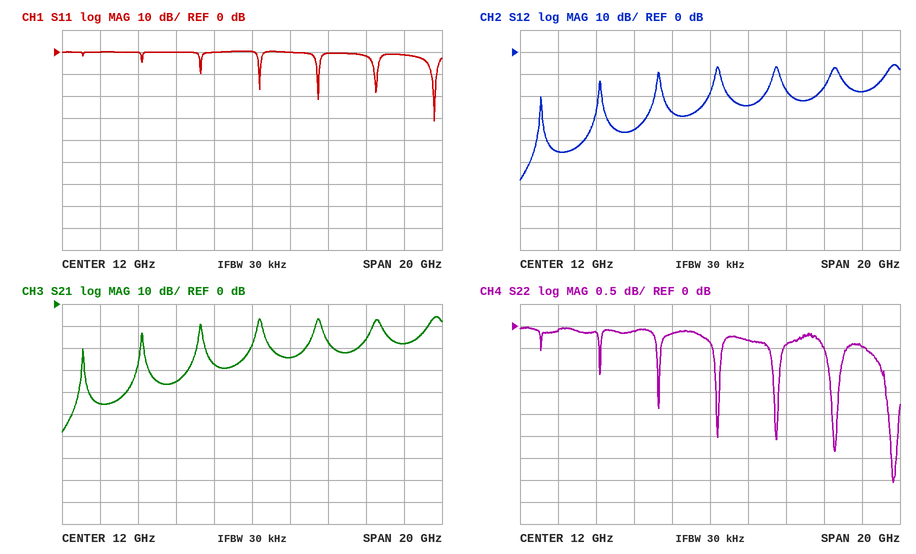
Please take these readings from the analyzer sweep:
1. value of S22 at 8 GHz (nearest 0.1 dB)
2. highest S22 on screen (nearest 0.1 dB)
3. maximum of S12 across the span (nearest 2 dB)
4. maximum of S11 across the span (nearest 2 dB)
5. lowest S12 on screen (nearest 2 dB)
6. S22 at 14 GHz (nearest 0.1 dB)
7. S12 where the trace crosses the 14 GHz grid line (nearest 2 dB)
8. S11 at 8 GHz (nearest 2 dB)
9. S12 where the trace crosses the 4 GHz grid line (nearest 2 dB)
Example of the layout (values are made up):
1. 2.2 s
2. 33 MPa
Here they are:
1. -0.1 dB
2. 0.0 dB
3. -6 dB
4. 0 dB
5. -58 dB
6. -0.3 dB
7. -24 dB
8. 0 dB
9. -46 dB
